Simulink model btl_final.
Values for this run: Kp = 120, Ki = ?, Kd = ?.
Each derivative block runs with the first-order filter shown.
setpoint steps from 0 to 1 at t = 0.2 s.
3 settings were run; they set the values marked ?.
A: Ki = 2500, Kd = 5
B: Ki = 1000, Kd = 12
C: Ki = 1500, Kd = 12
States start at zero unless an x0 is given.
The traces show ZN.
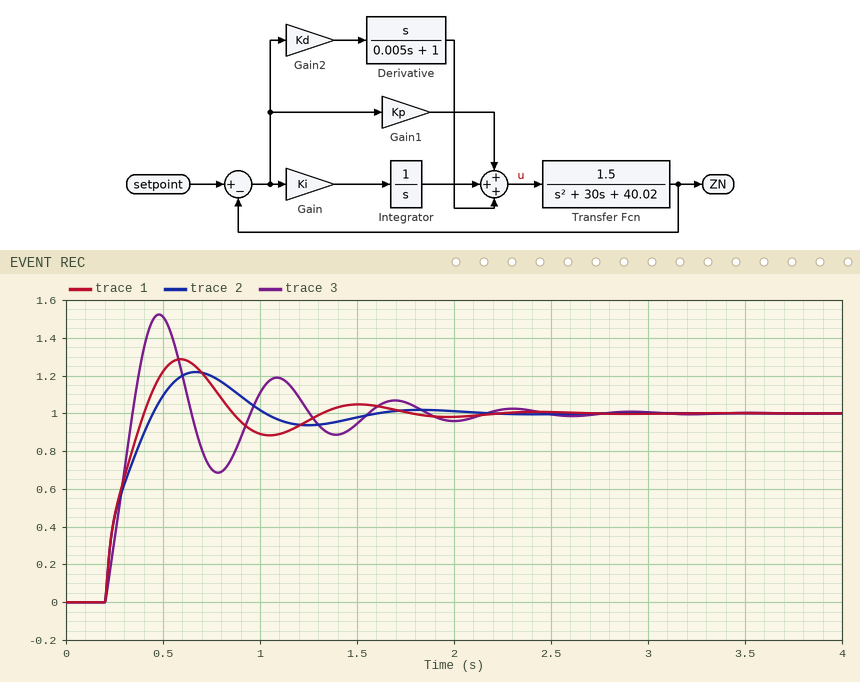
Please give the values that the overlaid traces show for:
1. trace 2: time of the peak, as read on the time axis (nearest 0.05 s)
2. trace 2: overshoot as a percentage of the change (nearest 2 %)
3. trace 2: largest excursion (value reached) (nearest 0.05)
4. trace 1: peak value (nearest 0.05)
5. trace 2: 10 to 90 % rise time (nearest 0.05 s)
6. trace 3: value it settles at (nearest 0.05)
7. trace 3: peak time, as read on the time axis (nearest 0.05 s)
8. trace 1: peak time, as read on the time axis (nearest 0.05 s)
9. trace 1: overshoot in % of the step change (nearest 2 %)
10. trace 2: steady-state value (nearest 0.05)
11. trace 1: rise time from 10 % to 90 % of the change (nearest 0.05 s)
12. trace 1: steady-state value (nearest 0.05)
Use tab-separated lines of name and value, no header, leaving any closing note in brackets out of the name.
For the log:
trace 2: time of the peak, as read on the time axis	0.65 s
trace 2: overshoot as a percentage of the change	22 %
trace 2: largest excursion (value reached)	1.20
trace 1: peak value	1.30
trace 2: 10 to 90 % rise time	0.20 s
trace 3: value it settles at	1.00
trace 3: peak time, as read on the time axis	0.50 s
trace 1: peak time, as read on the time axis	0.60 s
trace 1: overshoot in % of the step change	28 %
trace 2: steady-state value	1.00
trace 1: rise time from 10 % to 90 % of the change	0.15 s
trace 1: steady-state value	1.00
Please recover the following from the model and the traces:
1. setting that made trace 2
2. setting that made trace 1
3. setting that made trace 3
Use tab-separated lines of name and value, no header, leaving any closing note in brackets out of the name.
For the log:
setting that made trace 2	B
setting that made trace 1	C
setting that made trace 3	A
